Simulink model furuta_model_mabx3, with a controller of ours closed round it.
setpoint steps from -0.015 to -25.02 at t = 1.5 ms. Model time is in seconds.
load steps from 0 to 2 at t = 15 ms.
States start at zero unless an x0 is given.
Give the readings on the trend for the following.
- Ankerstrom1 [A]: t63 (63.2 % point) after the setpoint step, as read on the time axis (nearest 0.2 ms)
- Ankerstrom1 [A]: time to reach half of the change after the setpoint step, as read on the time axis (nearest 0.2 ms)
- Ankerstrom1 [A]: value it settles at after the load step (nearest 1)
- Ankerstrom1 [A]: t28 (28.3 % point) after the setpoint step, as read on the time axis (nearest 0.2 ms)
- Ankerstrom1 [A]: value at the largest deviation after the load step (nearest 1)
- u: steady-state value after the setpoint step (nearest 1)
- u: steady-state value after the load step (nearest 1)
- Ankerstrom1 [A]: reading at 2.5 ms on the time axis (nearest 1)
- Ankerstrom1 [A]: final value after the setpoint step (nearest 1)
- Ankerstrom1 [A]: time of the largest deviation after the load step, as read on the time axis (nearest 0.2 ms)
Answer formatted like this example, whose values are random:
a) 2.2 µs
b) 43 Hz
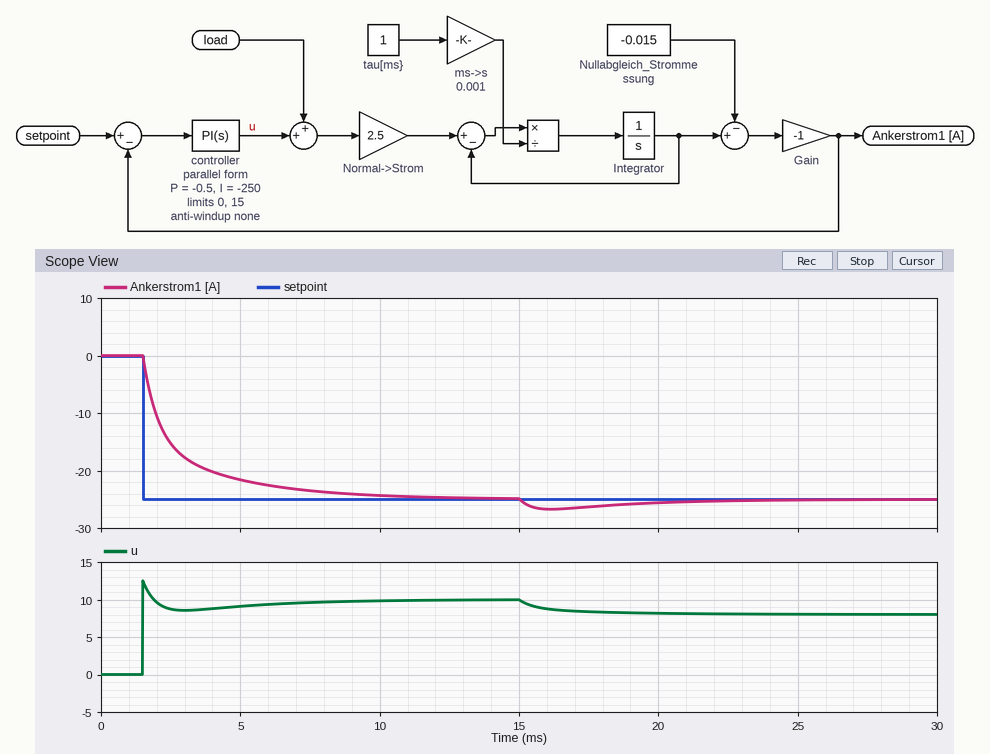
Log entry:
a) 2.6 ms
b) 2.2 ms
c) -25
d) 1.8 ms
e) -27
f) 10
g) 8
h) -15
i) -25
j) 16.2 ms
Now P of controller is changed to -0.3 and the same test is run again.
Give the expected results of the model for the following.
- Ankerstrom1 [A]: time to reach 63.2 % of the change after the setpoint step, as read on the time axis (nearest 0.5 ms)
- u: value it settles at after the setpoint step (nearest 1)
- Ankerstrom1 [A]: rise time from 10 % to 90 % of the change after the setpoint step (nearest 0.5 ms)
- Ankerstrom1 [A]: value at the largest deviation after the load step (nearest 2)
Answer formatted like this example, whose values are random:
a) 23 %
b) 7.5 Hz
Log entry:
a) 3.0 ms
b) 10
c) 3.5 ms
d) -28
